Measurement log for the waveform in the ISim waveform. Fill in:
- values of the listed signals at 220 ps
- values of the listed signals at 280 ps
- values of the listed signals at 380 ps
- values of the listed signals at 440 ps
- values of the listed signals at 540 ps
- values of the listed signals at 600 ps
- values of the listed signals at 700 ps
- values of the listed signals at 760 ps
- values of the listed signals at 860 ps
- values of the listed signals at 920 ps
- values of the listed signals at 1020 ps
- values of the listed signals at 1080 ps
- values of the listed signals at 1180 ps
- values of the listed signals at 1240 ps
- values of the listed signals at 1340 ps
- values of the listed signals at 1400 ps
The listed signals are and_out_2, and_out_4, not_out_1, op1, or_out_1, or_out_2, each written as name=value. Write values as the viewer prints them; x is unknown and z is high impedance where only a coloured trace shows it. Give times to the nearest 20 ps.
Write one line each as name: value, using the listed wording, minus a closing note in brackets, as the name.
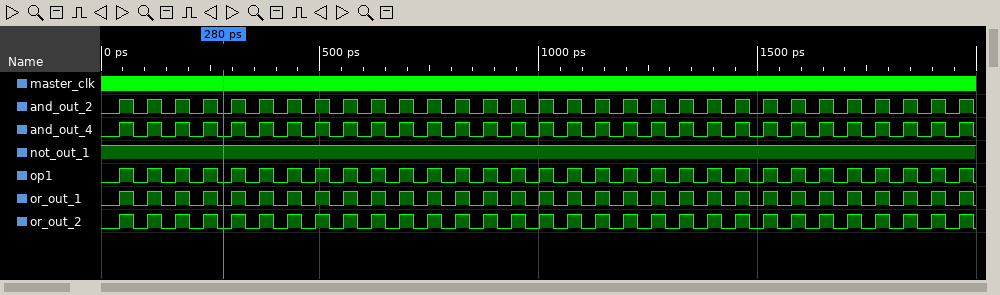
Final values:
values of the listed signals at 220 ps: and_out_2=0, and_out_4=0, not_out_1=1, op1=0, or_out_1=0, or_out_2=0
values of the listed signals at 280 ps: and_out_2=0, and_out_4=0, not_out_1=1, op1=0, or_out_1=0, or_out_2=0
values of the listed signals at 380 ps: and_out_2=1, and_out_4=1, not_out_1=1, op1=1, or_out_1=1, or_out_2=1
values of the listed signals at 440 ps: and_out_2=1, and_out_4=1, not_out_1=1, op1=1, or_out_1=1, or_out_2=1
values of the listed signals at 540 ps: and_out_2=0, and_out_4=0, not_out_1=1, op1=0, or_out_1=0, or_out_2=0
values of the listed signals at 600 ps: and_out_2=0, and_out_4=0, not_out_1=1, op1=0, or_out_1=0, or_out_2=0
values of the listed signals at 700 ps: and_out_2=1, and_out_4=1, not_out_1=1, op1=1, or_out_1=1, or_out_2=1
values of the listed signals at 760 ps: and_out_2=1, and_out_4=1, not_out_1=1, op1=1, or_out_1=1, or_out_2=1
values of the listed signals at 860 ps: and_out_2=0, and_out_4=0, not_out_1=1, op1=0, or_out_1=0, or_out_2=0
values of the listed signals at 920 ps: and_out_2=0, and_out_4=0, not_out_1=1, op1=0, or_out_1=0, or_out_2=0
values of the listed signals at 1020 ps: and_out_2=1, and_out_4=1, not_out_1=1, op1=1, or_out_1=1, or_out_2=1
values of the listed signals at 1080 ps: and_out_2=1, and_out_4=1, not_out_1=1, op1=1, or_out_1=1, or_out_2=1
values of the listed signals at 1180 ps: and_out_2=0, and_out_4=0, not_out_1=1, op1=0, or_out_1=0, or_out_2=0
values of the listed signals at 1240 ps: and_out_2=0, and_out_4=0, not_out_1=1, op1=0, or_out_1=0, or_out_2=0
values of the listed signals at 1340 ps: and_out_2=1, and_out_4=1, not_out_1=1, op1=1, or_out_1=1, or_out_2=1
values of the listed signals at 1400 ps: and_out_2=1, and_out_4=1, not_out_1=1, op1=1, or_out_1=1, or_out_2=1
